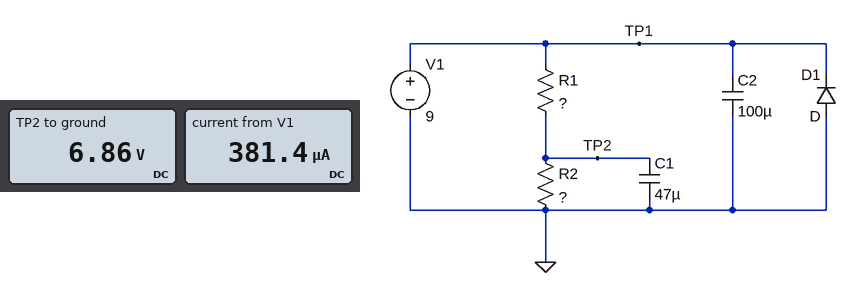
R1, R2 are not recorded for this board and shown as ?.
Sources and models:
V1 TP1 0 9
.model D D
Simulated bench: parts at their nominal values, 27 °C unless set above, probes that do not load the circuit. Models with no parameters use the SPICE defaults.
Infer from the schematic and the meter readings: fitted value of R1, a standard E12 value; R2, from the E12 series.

5.6 kΩ
18 kΩ
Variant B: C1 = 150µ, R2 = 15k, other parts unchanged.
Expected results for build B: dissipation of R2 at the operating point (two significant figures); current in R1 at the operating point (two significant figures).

2.9 mW
440 µA
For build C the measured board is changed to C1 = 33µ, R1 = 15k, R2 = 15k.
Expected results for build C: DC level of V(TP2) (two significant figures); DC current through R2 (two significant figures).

4.5 V
300 µA
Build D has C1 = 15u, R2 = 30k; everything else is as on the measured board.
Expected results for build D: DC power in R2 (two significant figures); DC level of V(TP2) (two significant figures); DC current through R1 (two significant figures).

1.9 mW
7.6 V
250 µA
